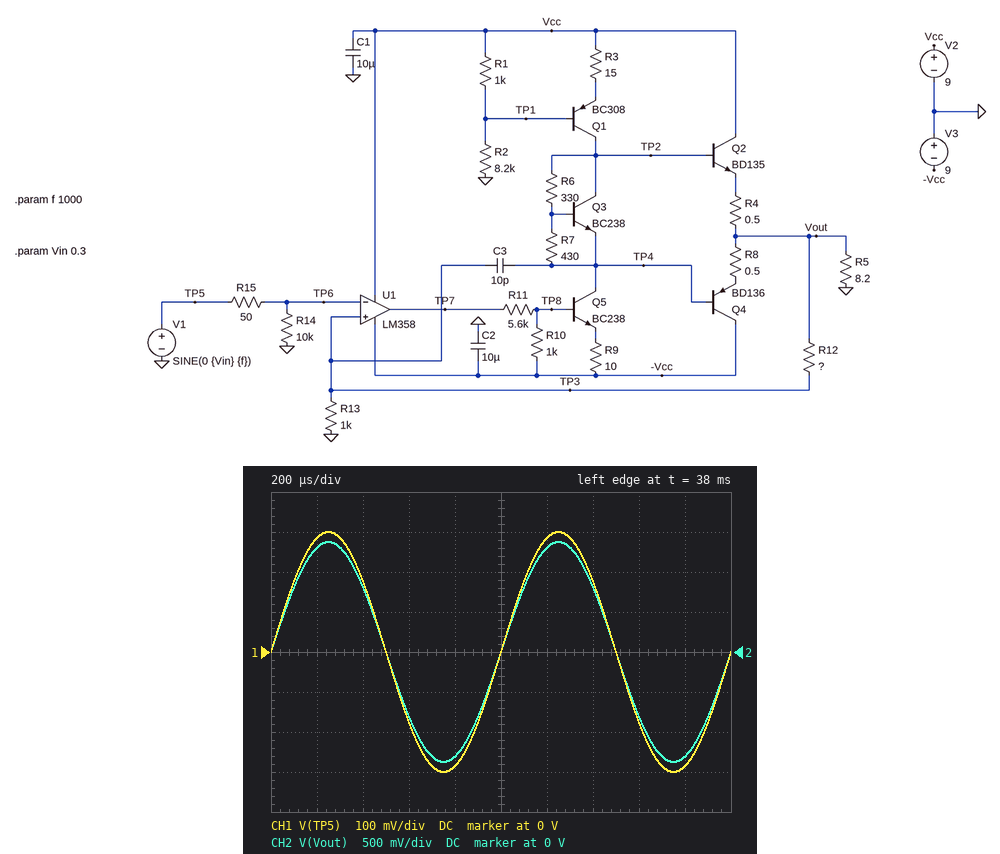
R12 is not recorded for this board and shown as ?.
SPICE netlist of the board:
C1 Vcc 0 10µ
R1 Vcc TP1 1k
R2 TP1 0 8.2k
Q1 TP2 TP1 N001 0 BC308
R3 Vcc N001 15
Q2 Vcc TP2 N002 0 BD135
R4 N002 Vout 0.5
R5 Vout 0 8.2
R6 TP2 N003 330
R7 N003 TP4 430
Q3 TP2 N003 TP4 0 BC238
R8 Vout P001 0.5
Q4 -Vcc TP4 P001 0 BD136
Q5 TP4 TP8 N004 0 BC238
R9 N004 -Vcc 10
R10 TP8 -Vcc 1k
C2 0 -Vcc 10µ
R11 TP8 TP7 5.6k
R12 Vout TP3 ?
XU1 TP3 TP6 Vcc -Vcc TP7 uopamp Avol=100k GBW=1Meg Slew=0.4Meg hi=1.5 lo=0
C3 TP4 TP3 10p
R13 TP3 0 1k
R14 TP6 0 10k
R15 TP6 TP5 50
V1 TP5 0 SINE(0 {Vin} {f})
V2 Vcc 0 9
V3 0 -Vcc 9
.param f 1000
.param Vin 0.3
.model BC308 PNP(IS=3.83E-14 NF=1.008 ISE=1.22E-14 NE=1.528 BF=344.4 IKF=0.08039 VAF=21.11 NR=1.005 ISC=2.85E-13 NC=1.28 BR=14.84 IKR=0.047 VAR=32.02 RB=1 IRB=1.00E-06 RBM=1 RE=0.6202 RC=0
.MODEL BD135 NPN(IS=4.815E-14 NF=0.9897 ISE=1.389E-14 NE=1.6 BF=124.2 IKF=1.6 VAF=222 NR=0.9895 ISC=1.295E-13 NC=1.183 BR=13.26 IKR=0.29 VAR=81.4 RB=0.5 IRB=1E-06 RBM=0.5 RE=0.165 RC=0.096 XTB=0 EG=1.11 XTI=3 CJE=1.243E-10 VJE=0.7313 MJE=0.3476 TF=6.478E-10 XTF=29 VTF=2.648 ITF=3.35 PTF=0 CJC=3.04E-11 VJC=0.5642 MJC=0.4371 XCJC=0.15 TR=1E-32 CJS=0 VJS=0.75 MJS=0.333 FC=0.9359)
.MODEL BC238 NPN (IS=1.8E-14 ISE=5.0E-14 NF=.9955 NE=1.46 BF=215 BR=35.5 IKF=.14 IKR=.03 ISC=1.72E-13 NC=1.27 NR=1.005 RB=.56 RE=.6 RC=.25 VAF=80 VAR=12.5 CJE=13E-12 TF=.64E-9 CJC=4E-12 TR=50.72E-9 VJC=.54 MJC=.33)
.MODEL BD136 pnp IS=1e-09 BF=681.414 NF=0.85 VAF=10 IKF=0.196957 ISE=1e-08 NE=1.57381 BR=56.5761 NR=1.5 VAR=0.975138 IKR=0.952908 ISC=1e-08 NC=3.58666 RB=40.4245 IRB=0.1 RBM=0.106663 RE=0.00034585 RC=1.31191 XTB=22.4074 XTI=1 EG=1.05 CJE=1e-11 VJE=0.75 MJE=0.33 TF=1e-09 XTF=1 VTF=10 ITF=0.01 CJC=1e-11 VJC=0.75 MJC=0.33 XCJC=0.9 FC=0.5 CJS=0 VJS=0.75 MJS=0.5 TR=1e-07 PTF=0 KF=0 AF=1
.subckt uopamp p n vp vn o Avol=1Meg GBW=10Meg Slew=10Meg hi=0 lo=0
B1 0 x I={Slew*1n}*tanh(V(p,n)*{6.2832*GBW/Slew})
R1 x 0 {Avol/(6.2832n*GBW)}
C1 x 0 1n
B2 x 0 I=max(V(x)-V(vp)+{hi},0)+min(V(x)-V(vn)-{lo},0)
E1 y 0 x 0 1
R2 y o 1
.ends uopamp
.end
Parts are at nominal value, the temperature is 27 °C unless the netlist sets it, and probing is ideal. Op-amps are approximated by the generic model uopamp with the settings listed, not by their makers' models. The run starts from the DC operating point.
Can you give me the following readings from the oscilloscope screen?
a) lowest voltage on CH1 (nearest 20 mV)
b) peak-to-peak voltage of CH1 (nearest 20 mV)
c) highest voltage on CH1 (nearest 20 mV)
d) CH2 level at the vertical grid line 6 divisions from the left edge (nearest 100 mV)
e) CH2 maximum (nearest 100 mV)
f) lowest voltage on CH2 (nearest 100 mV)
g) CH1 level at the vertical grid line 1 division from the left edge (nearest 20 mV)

-300 mV
600 mV
300 mV
1.3 V
1.4 V
-1.4 V
280 mV
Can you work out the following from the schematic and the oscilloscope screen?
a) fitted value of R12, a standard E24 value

3.6 kΩ
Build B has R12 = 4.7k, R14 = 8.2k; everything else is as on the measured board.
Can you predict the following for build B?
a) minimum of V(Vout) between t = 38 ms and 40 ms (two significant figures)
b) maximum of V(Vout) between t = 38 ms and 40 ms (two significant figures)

-1.7 V
1.7 V
